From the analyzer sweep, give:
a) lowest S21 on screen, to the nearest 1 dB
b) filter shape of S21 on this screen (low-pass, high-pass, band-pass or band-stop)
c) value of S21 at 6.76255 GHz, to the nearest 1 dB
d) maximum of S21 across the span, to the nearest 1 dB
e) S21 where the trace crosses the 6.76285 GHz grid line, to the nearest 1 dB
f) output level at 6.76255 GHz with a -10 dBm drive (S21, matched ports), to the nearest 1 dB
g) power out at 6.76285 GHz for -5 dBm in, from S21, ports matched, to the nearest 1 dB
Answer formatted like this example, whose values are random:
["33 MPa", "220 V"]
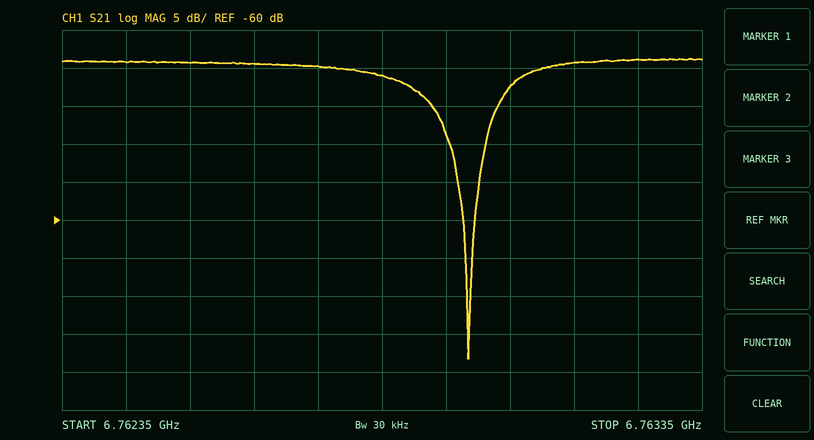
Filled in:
["-78 dB", "band-stop", "-39 dB", "-39 dB", "-41 dB", "-49 dBm", "-46 dBm"]
